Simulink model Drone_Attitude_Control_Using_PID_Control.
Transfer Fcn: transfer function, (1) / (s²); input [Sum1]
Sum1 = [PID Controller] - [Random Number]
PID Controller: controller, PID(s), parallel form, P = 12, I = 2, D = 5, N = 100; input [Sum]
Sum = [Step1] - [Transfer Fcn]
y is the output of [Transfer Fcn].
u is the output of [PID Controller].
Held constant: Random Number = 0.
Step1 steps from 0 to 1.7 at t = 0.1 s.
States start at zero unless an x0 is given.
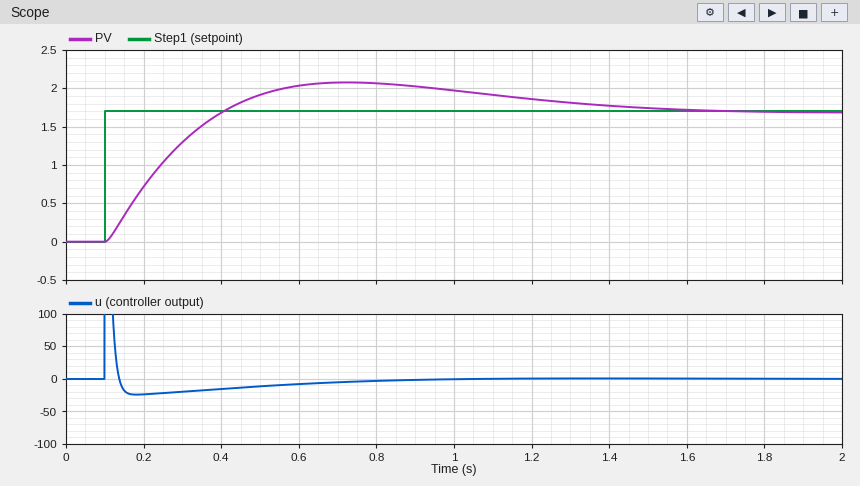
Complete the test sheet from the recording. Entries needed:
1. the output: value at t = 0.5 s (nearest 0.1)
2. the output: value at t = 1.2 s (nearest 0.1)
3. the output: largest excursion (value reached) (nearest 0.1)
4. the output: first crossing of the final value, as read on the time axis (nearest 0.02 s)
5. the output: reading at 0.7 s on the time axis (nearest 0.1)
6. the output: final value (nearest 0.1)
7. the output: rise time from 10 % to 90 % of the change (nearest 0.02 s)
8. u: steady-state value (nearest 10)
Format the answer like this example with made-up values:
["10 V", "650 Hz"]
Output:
["1.9", "1.9", "2.1", "0.40 s", "2.1", "1.7", "0.22 s", "0"]
